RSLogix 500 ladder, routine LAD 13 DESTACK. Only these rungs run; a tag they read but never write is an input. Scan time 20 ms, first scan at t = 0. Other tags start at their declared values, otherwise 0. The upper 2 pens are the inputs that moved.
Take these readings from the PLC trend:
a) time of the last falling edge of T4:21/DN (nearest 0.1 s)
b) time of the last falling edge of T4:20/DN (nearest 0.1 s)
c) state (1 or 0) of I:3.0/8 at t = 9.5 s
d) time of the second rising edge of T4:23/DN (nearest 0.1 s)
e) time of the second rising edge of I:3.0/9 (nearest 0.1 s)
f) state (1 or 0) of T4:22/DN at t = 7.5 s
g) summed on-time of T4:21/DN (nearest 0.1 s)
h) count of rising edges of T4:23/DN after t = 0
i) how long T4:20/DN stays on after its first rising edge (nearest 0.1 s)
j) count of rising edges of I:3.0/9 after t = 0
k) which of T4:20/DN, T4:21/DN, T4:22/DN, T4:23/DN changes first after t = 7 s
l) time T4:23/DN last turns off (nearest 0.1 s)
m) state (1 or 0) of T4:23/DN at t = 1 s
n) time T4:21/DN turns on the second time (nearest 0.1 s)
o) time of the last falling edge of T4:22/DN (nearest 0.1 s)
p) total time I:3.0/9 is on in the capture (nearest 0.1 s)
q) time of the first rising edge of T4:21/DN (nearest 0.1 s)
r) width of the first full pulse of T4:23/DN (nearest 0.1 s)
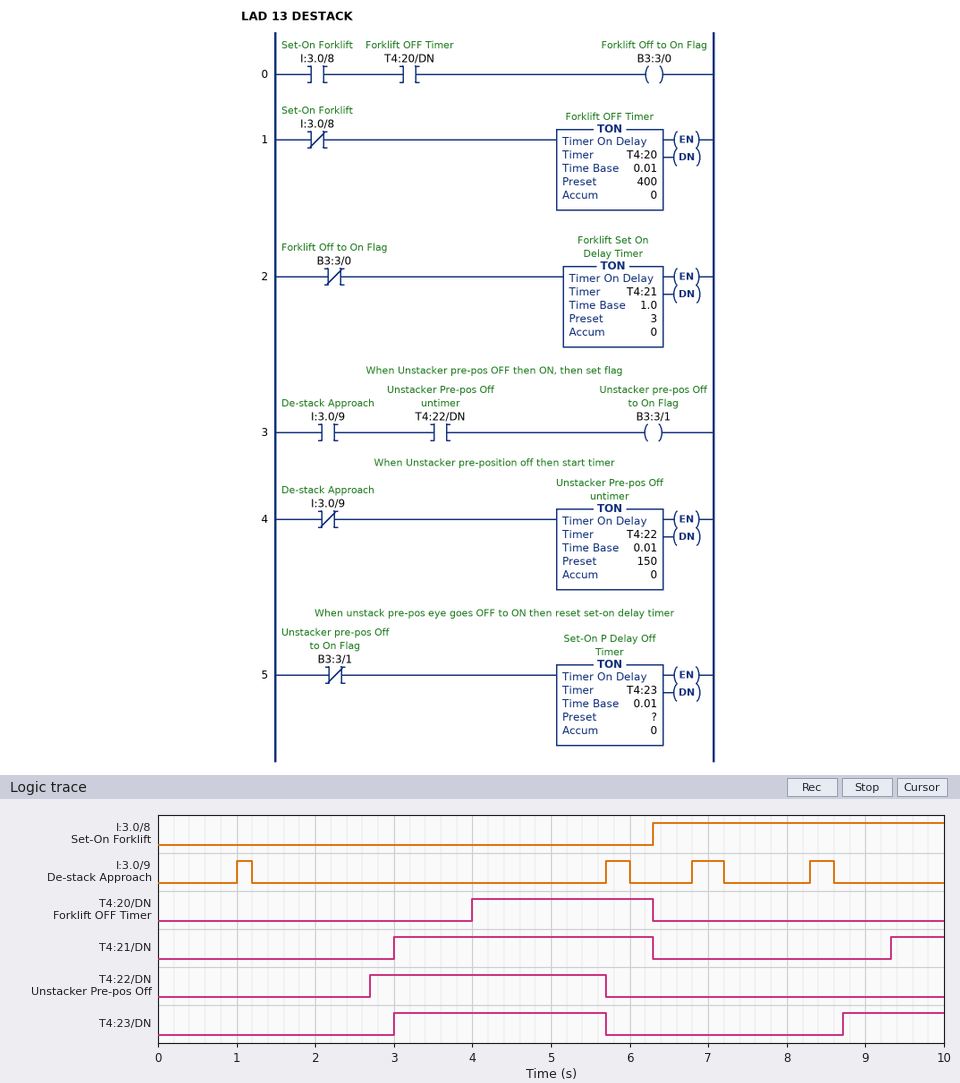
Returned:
6.3 s
6.3 s
1
8.7 s
5.7 s
0
4.0 s
2
2.3 s
4
T4:23/DN
5.7 s
0
9.3 s
5.7 s
1.2 s
3.0 s
2.7 s
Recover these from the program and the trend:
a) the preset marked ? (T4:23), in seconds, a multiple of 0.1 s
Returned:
3.0 s
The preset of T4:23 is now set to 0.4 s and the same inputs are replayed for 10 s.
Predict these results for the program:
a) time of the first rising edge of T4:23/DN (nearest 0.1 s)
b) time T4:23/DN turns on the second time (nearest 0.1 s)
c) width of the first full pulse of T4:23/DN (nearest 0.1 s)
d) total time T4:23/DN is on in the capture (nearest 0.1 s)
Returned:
0.4 s
6.1 s
5.3 s
9.2 s
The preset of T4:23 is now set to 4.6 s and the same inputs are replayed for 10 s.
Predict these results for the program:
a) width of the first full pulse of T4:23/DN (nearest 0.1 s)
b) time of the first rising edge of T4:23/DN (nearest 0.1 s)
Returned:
1.1 s
4.6 s
